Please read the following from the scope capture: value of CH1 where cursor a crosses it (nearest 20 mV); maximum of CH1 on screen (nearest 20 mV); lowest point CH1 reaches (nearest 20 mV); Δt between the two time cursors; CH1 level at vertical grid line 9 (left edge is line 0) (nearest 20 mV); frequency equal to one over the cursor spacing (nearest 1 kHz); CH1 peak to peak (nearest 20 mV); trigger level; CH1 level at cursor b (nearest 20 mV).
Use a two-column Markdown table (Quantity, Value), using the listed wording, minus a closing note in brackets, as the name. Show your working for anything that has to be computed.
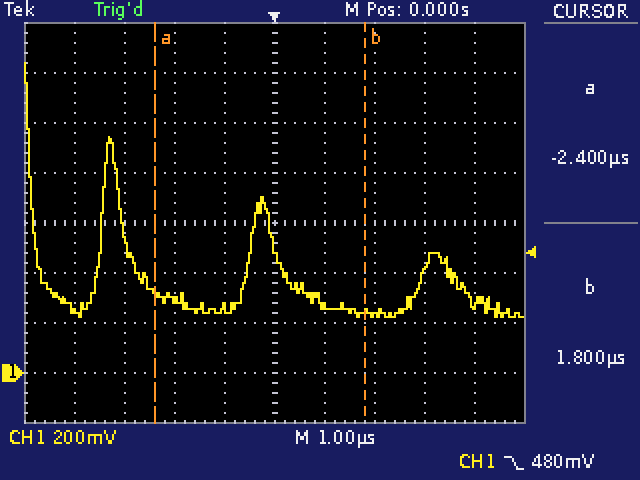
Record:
| Quantity | Value |
|---|---|
| value of CH1 where cursor a crosses it | 320 mV |
| maximum of CH1 on screen | 1.24 V |
| lowest point CH1 reaches | 220 mV |
| Δt between the two time cursors | 1.8 µs − (-2.4 µs) = 4.2 µs |
| CH1 level at vertical grid line 9 (left edge is line 0) | 280 mV |
| frequency equal to one over the cursor spacing | 1 / 4.2 µs ≈ 238 kHz |
| CH1 peak to peak | 1.24 V − (220 mV) = 1.02 V |
| trigger level | 480 mV |
| CH1 level at cursor b | 240 mV |
